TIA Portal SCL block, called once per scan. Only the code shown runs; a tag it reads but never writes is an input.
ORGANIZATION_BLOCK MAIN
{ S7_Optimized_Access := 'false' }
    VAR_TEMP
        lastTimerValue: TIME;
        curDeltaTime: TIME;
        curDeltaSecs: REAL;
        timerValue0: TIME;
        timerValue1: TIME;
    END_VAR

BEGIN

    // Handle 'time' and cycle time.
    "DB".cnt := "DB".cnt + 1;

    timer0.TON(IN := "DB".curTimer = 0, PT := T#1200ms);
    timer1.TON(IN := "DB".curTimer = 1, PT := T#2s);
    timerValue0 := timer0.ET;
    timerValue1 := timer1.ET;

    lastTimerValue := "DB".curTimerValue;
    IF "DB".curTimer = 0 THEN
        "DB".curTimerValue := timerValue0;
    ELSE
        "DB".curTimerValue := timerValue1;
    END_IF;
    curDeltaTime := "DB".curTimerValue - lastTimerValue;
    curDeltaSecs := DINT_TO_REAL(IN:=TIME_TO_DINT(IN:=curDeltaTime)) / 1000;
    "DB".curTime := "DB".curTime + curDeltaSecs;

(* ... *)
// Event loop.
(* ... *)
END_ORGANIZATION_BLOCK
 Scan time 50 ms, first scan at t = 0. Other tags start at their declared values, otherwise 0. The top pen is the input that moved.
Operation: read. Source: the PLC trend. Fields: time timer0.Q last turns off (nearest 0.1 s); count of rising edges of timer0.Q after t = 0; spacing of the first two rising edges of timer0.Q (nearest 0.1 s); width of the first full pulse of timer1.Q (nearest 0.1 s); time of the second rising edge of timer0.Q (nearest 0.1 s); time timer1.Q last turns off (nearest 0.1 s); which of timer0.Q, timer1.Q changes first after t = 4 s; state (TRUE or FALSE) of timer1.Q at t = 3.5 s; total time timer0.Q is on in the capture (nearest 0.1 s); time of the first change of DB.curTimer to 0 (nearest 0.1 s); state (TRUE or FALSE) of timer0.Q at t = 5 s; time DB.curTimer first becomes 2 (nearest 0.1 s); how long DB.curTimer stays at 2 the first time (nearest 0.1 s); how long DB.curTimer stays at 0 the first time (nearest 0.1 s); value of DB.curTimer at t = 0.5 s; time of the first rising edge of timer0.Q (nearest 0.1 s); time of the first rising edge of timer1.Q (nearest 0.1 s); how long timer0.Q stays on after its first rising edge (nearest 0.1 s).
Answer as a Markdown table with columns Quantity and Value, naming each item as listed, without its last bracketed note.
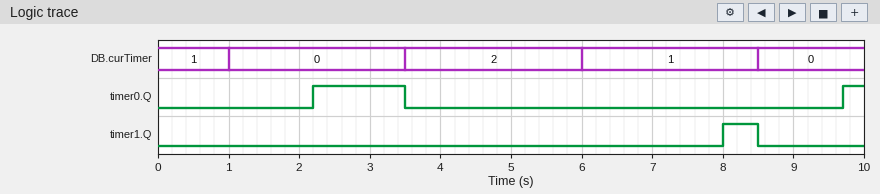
| Quantity | Value |
|---|---|
| time timer0.Q last turns off | 3.5 s |
| count of rising edges of timer0.Q after t = 0 | 2 |
| spacing of the first two rising edges of timer0.Q | 7.5 s |
| width of the first full pulse of timer1.Q | 0.5 s |
| time of the second rising edge of timer0.Q | 9.7 s |
| time timer1.Q last turns off | 8.5 s |
| which of timer0.Q, timer1.Q changes first after t = 4 s | timer1.Q |
| state (TRUE or FALSE) of timer1.Q at t = 3.5 s | FALSE |
| total time timer0.Q is on in the capture | 1.6 s |
| time of the first change of DB.curTimer to 0 | 1.0 s |
| state (TRUE or FALSE) of timer0.Q at t = 5 s | FALSE |
| time DB.curTimer first becomes 2 | 3.5 s |
| how long DB.curTimer stays at 2 the first time | 2.5 s |
| how long DB.curTimer stays at 0 the first time | 2.5 s |
| value of DB.curTimer at t = 0.5 s | 1 |
| time of the first rising edge of timer0.Q | 2.2 s |
| time of the first rising edge of timer1.Q | 8.0 s |
| how long timer0.Q stays on after its first rising edge | 1.3 s |
